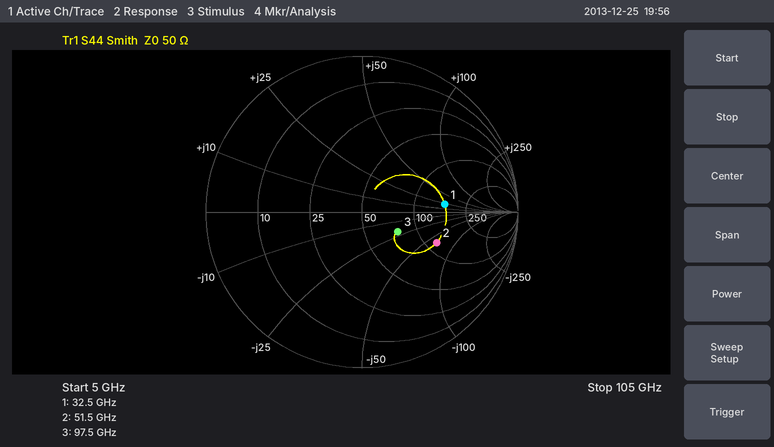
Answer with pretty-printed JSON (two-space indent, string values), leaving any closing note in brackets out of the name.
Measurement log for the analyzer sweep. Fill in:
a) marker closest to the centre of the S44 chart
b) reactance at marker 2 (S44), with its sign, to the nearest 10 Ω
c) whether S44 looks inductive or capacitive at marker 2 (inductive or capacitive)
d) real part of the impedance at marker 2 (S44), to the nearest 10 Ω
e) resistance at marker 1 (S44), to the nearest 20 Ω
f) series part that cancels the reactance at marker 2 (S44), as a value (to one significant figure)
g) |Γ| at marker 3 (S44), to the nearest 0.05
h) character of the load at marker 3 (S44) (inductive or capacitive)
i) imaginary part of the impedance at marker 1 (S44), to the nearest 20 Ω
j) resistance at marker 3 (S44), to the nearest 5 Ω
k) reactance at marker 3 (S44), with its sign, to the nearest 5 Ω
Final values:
{
  "marker closest to the centre of the S44 chart": "marker 3",
  "reactance at marker 2 (S44), with its sign, to the nearest 10 Ω": "-60 Ω",
  "whether S44 looks inductive or capacitive at marker 2": "capacitive",
  "real part of the impedance at marker 2 (S44), to the nearest 10 Ω": "120 Ω",
  "resistance at marker 1 (S44), to the nearest 20 Ω": "160 Ω",
  "series part that cancels the reactance at marker 2 (S44), as a value": "200 pH",
  "|Γ| at marker 3 (S44), to the nearest 0.05": "0.25",
  "character of the load at marker 3 (S44)": "capacitive",
  "imaginary part of the impedance at marker 1 (S44), to the nearest 20 Ω": "+20 Ω",
  "resistance at marker 3 (S44), to the nearest 5 Ω": "75 Ω",
  "reactance at marker 3 (S44), with its sign, to the nearest 5 Ω": "-20 Ω"
}
